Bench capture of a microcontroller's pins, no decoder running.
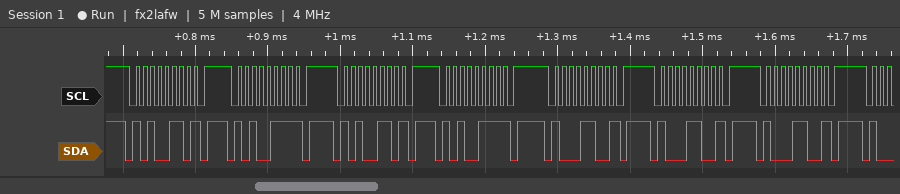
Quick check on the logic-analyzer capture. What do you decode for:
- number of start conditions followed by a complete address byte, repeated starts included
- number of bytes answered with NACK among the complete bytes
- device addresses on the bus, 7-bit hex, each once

7
7
0x53 0x46
